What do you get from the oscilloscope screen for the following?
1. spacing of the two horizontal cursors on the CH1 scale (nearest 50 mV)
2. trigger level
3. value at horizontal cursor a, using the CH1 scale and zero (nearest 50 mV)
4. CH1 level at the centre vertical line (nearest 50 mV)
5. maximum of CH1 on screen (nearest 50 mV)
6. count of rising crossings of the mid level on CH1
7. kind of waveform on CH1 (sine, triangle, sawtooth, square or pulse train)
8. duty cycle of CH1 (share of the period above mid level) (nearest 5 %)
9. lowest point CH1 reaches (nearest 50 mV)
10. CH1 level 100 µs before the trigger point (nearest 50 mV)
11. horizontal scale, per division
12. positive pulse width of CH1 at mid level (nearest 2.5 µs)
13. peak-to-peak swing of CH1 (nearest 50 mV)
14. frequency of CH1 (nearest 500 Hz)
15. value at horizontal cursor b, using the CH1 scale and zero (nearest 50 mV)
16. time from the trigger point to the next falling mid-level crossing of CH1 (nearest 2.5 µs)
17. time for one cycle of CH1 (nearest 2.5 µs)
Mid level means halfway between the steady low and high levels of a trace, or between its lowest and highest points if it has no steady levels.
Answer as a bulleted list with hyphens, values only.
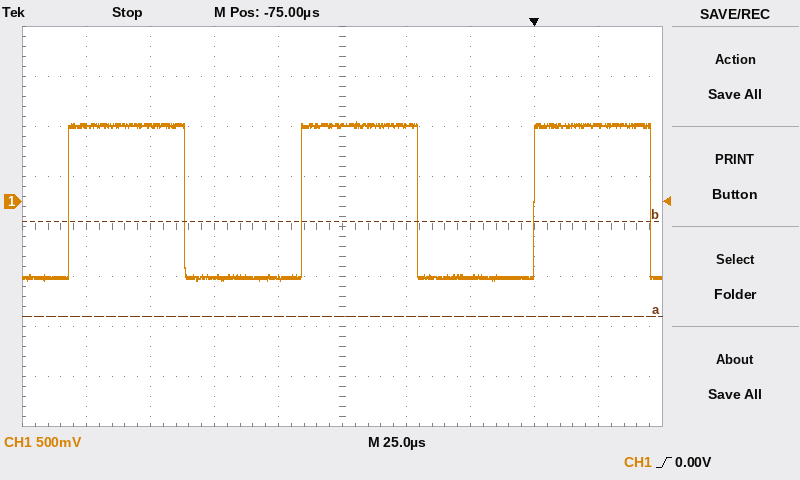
- 950 mV
- 0.00 V
- -1.15 V
- 750 mV
- 800 mV
- 3
- square
- 50 %
- -800 mV
- -750 mV
- 25 µs
- 45.0 µs
- 1.60 V
- 11.0 kHz
- -200 mV
- 45.0 µs
- 90.0 µs
